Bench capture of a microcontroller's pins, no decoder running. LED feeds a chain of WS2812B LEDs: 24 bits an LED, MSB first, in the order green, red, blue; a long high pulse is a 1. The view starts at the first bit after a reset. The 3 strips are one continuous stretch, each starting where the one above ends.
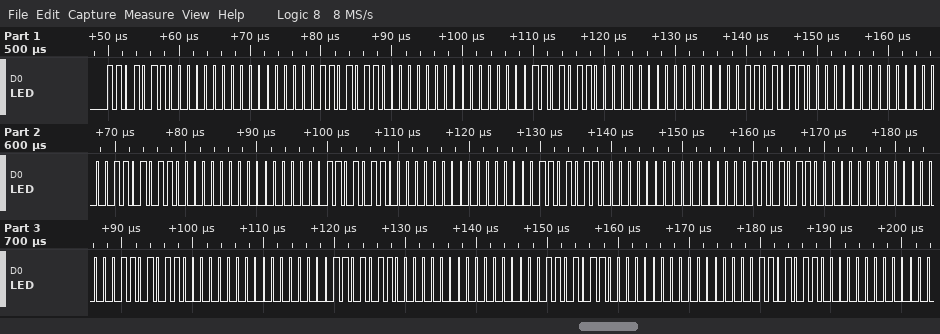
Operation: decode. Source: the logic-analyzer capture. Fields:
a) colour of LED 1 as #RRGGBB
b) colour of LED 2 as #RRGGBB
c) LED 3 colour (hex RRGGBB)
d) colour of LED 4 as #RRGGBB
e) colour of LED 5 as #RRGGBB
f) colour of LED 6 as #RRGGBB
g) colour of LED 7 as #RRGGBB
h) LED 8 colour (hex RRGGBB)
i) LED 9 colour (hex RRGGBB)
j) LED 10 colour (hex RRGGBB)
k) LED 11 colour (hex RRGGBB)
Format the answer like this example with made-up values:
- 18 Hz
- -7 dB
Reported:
- #00D600
- #00D600
- #00D600
- #00D600
- #00D600
- #00D600
- #00D600
- #00D600
- #00D600
- #00D600
- #00D600
